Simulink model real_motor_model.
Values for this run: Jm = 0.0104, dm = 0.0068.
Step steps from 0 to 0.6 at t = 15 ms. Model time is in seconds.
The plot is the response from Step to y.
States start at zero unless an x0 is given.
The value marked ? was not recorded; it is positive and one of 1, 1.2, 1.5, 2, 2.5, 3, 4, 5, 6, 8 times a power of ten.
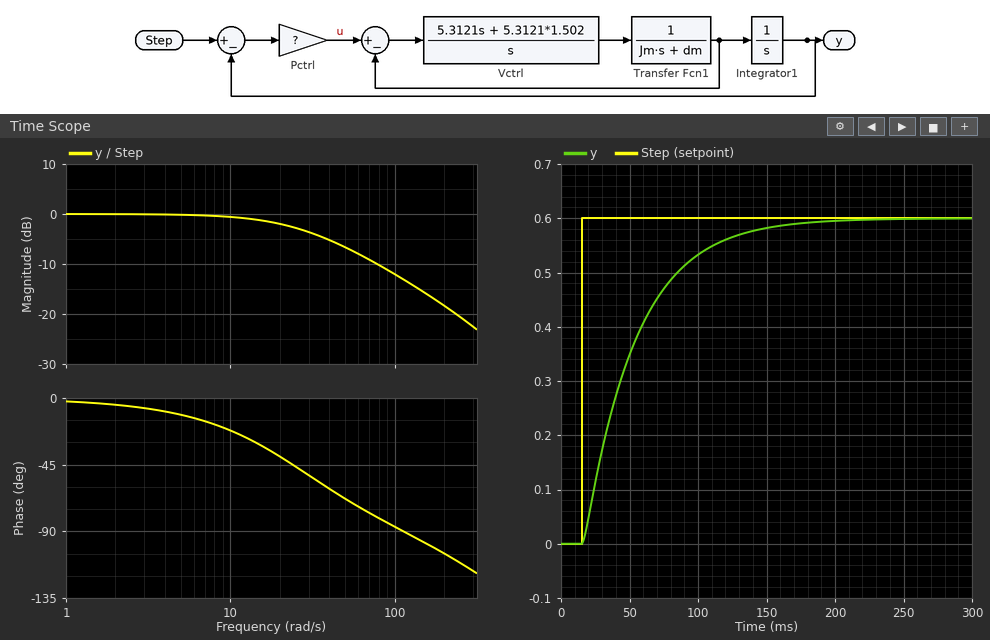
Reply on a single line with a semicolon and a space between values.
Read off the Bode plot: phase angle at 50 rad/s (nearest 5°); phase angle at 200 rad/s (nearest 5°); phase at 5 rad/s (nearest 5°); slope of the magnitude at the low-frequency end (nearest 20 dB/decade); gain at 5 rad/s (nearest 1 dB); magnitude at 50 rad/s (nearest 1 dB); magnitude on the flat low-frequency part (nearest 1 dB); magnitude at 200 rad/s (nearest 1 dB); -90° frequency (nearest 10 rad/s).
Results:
-70°; -105°; -10°; 0 dB/decade; 0 dB; -7 dB; 0 dB; -18 dB; 110 rad/s
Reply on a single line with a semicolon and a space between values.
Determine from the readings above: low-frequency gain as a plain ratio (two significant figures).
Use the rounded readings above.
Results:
1.0
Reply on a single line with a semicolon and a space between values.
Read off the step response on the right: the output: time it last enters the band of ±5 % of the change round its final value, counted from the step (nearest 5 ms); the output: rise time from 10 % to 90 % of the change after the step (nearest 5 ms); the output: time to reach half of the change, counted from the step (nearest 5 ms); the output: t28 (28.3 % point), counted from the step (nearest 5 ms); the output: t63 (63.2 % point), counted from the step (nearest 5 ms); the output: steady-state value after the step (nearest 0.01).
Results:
115 ms; 85 ms; 30 ms; 15 ms; 40 ms; 0.60
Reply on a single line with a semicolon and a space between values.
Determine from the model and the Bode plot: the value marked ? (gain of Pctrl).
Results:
25
